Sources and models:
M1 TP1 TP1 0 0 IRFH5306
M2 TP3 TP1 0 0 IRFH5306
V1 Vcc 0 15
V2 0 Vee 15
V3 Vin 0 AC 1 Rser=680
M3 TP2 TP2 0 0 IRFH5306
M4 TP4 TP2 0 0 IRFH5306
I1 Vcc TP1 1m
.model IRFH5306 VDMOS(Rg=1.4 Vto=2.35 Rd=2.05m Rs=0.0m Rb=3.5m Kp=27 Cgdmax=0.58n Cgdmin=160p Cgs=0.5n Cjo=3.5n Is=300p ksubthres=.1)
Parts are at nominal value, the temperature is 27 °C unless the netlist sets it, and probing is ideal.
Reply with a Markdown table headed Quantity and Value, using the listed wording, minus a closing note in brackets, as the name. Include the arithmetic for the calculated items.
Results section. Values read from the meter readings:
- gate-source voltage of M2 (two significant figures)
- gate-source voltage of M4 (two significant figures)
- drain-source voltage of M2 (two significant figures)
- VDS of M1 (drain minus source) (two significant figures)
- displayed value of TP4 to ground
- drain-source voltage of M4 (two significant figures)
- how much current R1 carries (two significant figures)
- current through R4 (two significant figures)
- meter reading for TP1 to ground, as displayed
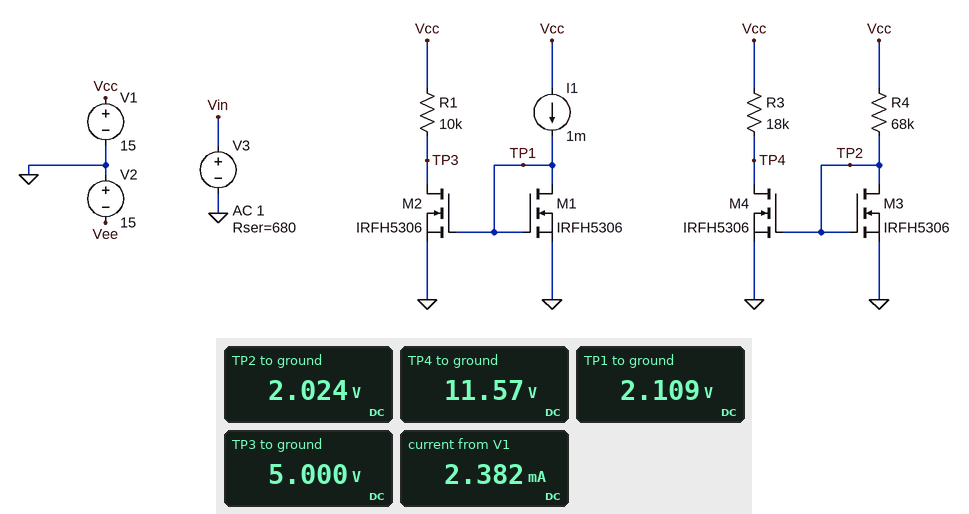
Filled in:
| Quantity | Value |
|---|---|
| gate-source voltage of M2 | 2.109 V = 2.1 V |
| gate-source voltage of M4 | 2.024 V = 2.0 V |
| drain-source voltage of M2 | 5 V = 5.0 V |
| VDS of M1 (drain minus source) | 2.109 V = 2.1 V |
| displayed value of TP4 to ground | 11.57 V |
| drain-source voltage of M4 | 11.57 V = 12 V |
| how much current R1 carries | (15 V - 5 V) / 10 kΩ = 1.0 mA |
| current through R4 | (15 V - 2.024 V) / 68 kΩ = 190 µA |
| meter reading for TP1 to ground, as displayed | 2.109 V |
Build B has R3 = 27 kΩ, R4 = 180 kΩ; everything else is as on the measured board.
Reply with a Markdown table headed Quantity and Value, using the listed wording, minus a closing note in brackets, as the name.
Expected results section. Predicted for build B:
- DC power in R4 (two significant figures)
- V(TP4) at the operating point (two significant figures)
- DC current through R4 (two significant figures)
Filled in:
| Quantity | Value |
|---|---|
| DC power in R4 | 940 µW |
| V(TP4) at the operating point | 13 V |
| DC current through R4 | 72 µA |
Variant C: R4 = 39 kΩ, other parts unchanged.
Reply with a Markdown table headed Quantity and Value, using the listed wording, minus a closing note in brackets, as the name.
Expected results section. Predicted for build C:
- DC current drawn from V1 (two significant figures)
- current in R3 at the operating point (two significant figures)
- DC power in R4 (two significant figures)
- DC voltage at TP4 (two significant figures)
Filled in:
| Quantity | Value |
|---|---|
| DC current drawn from V1 | 2.7 mA |
| current in R3 at the operating point | 330 µA |
| DC power in R4 | 4.3 mW |
| DC voltage at TP4 | 9.0 V |
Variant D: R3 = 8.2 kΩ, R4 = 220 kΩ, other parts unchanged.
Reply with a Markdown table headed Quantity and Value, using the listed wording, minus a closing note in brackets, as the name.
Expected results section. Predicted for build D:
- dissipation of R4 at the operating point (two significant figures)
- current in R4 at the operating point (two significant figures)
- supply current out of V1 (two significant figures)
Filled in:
| Quantity | Value |
|---|---|
| dissipation of R4 at the operating point | 770 µW |
| current in R4 at the operating point | 59 µA |
| supply current out of V1 | 2.1 mA |
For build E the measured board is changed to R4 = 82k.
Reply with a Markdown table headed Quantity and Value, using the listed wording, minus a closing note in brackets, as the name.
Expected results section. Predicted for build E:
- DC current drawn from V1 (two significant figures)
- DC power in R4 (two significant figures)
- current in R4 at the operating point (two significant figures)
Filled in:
| Quantity | Value |
|---|---|
| DC current drawn from V1 | 2.3 mA |
| DC power in R4 | 2.1 mW |
| current in R4 at the operating point | 160 µA |
